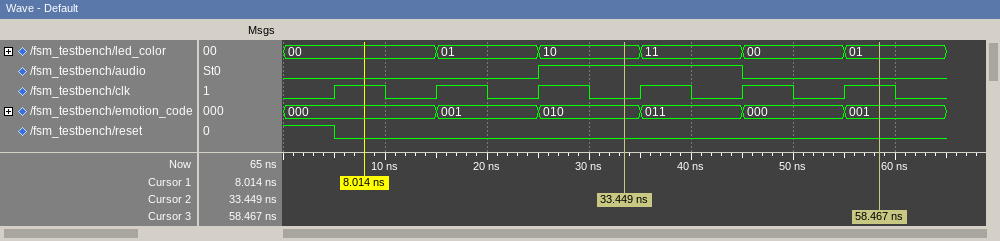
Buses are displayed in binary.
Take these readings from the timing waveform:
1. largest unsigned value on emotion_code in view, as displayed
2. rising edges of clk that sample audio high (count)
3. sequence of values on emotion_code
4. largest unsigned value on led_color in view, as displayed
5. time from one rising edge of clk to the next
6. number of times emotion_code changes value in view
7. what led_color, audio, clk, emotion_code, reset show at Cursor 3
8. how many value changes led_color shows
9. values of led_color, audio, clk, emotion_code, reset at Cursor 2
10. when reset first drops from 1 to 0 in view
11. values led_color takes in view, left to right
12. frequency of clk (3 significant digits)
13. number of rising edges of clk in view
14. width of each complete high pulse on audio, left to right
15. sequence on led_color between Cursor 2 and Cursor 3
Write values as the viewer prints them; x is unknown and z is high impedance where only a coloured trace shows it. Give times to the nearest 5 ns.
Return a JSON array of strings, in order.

["011", "2", "000, 001, 010, 011, 000, 001", "11", "10 ns", "5", "led_color=01, audio=0, clk=1, emotion_code=001, reset=0", "5", "led_color=10, audio=1, clk=0, emotion_code=010, reset=0", "5 ns", "00, 01, 10, 11, 00, 01", "100 MHz", "6", "20 ns", "10, 11, 00, 01"]
